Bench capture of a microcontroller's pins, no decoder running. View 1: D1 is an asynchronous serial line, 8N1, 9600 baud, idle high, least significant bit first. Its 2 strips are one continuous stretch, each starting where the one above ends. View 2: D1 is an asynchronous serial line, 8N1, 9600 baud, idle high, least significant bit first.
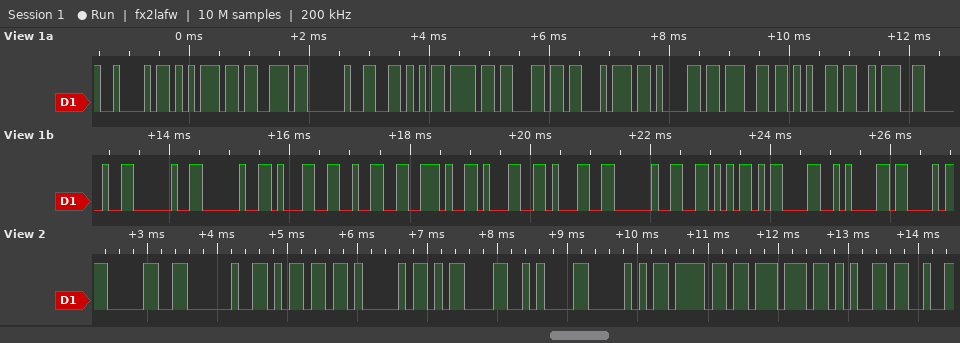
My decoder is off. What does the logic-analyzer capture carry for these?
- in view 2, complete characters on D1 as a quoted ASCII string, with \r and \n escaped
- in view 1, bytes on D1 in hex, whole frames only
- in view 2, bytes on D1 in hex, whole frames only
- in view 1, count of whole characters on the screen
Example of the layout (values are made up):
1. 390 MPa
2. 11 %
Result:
1. "0 mA\r\nPowe"
2. 42 75 73 20 56 6F 6C 74 61 67 65 3A 20 20 20 31 32 2E 31 31 20 56 0D 0A 43
3. 30 20 6D 41 0D 0A 50 6F 77 65
4. 25
